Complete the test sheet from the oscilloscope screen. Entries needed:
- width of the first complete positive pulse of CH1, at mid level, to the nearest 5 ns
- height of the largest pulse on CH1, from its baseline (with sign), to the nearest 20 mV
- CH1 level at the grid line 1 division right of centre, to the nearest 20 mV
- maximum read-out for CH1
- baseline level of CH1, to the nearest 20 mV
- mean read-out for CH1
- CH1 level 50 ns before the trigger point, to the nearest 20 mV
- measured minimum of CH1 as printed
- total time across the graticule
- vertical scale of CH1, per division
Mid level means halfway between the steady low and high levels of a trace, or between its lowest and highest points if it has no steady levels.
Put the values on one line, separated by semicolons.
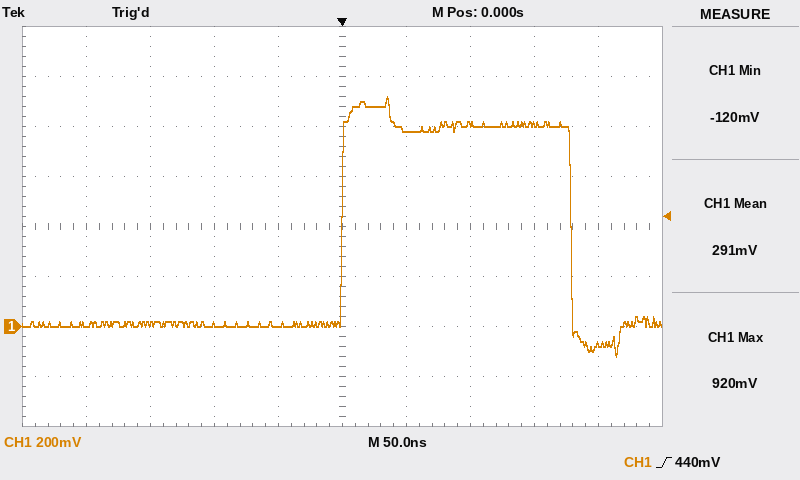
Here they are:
180 ns; +920 mV; 780 mV; 920 mV; 0 mV; 291 mV; 0 mV; -120 mV; 500 ns; 200 mV
